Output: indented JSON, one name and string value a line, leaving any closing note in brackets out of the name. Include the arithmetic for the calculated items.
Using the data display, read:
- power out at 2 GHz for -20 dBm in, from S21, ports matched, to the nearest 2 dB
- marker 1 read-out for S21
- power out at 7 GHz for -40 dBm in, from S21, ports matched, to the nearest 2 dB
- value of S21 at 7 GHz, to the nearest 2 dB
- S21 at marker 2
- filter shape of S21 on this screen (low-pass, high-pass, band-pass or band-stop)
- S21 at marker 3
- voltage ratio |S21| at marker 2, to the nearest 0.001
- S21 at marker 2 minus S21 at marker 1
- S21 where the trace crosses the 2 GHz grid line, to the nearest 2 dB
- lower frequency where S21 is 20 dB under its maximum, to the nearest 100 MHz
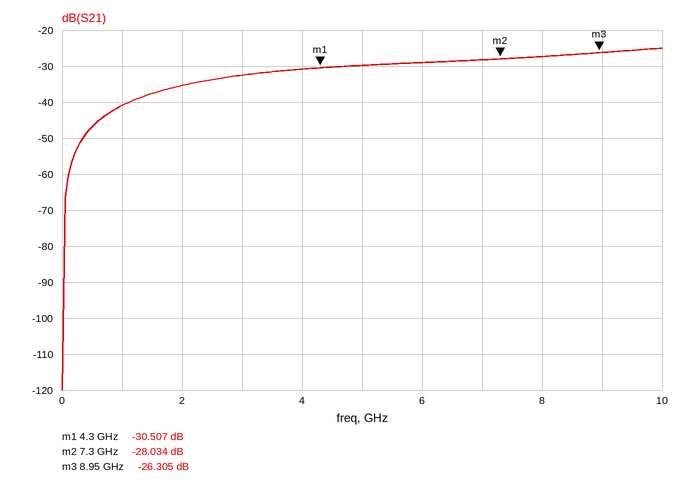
{
  "power out at 2 GHz for -20 dBm in, from S21, ports matched, to the nearest 2 dB": "-20 dBm + (-36 dB) = -56 dBm",
  "marker 1 read-out for S21": "-30.507 dB",
  "power out at 7 GHz for -40 dBm in, from S21, ports matched, to the nearest 2 dB": "-40 dBm + (-28 dB) = -68 dBm",
  "value of S21 at 7 GHz, to the nearest 2 dB": "-28 dB",
  "S21 at marker 2": "-28.034 dB",
  "filter shape of S21 on this screen": "high-pass",
  "S21 at marker 3": "-26.305 dB",
  "voltage ratio |S21| at marker 2, to the nearest 0.001": "10^(-28.034/20) ≈ 0.040",
  "S21 at marker 2 minus S21 at marker 1": "-28.034 − (-30.507) = 2.473 dB",
  "S21 where the trace crosses the 2 GHz grid line, to the nearest 2 dB": "-36 dB",
  "lower frequency where S21 is 20 dB under its maximum, to the nearest 100 MHz": "600 MHz"
}
